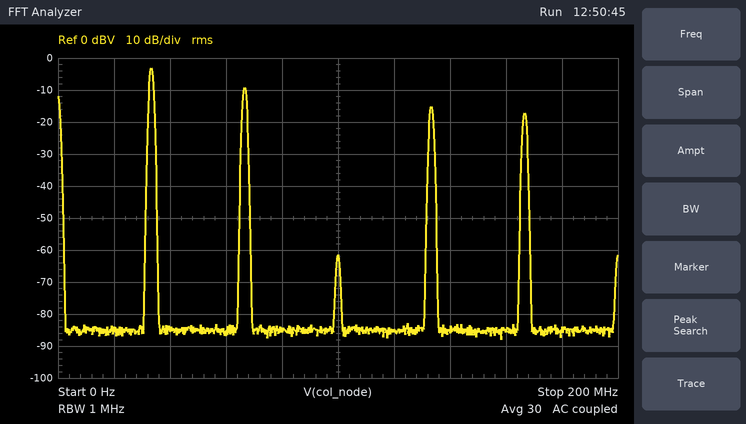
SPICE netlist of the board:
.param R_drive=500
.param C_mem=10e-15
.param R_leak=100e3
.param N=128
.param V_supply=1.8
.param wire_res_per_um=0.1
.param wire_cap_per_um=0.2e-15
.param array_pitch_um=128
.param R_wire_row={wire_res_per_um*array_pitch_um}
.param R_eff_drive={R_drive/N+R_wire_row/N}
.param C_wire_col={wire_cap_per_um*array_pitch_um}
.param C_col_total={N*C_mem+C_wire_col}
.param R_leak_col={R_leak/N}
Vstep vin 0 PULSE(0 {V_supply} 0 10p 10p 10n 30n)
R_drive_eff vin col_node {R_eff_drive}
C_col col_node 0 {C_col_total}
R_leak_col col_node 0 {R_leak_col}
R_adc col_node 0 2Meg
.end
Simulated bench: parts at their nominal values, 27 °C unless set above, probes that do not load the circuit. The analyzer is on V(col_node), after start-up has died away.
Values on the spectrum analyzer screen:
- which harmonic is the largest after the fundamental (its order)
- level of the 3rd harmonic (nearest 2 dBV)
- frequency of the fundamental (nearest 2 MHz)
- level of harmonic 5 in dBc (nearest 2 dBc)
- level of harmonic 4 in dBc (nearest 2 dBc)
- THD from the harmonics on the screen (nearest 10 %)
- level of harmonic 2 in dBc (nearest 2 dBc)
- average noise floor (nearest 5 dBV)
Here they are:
2
-62 dBV
34 MHz
-14 dBc
-12 dBc
60 %
-6 dBc
-85 dBV
